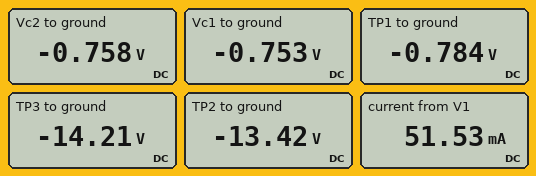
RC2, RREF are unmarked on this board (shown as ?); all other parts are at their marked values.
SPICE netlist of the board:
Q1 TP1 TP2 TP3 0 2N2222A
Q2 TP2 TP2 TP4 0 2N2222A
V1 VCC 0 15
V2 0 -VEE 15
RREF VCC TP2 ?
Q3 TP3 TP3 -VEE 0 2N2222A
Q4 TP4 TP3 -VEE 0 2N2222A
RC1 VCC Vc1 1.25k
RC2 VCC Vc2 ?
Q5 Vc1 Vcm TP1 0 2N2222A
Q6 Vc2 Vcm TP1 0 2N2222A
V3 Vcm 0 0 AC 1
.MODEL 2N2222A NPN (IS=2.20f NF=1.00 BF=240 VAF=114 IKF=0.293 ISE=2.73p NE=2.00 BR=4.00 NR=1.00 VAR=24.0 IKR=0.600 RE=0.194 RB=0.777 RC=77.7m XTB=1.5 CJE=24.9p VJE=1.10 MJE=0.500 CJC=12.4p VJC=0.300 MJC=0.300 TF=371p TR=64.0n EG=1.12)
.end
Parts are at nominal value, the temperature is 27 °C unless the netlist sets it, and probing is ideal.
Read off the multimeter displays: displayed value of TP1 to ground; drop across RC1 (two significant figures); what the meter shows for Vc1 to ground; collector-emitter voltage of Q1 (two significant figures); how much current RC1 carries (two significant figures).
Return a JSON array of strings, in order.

["-0.784 V", "16 V", "-0.753 V", "13 V", "13 mA"]
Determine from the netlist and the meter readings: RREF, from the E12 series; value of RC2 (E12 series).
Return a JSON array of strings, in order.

["1 kΩ", "1.5 kΩ"]
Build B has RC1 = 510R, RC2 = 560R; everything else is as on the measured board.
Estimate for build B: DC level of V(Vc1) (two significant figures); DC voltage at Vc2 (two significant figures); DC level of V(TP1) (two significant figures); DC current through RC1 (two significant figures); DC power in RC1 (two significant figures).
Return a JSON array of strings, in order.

["7.8 V", "7.1 V", "-770 mV", "14 mA", "100 mW"]
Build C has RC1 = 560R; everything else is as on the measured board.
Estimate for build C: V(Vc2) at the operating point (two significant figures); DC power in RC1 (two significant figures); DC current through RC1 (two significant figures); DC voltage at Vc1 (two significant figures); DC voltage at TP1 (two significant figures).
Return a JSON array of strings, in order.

["-730 mV", "160 mW", "17 mA", "5.7 V", "-770 mV"]
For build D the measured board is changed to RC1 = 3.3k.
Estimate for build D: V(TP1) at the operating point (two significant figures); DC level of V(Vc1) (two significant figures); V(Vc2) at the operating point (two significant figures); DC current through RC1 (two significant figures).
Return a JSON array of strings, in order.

["-800 mV", "-790 mV", "-780 mV", "4.8 mA"]
